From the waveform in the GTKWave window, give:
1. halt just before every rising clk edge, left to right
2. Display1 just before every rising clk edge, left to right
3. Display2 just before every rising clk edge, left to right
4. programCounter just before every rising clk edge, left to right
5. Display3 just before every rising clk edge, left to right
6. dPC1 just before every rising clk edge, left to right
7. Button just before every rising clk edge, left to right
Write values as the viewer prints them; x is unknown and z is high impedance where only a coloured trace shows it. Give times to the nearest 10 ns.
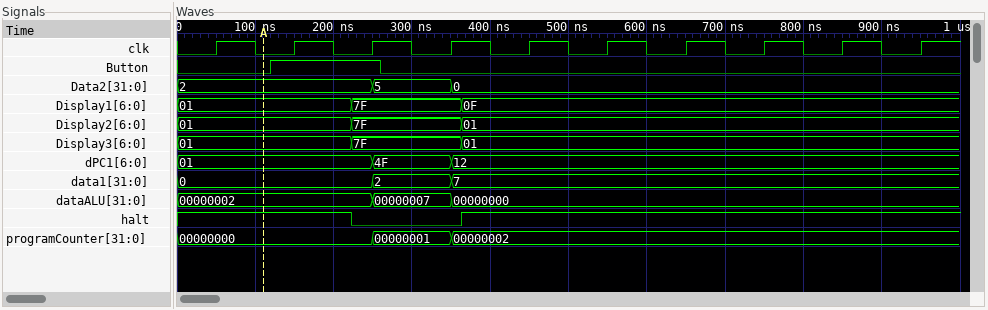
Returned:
1 1 0 0 1 1 1 1 1 1
01, 01, 7F, 7F, 0F, 0F, 0F, 0F, 0F, 0F
01, 01, 7F, 7F, 01, 01, 01, 01, 01, 01
00000000, 00000000, 00000000, 00000001, 00000002, 00000002, 00000002, 00000002, 00000002, 00000002
01, 01, 7F, 7F, 01, 01, 01, 01, 01, 01
01, 01, 01, 4F, 12, 12, 12, 12, 12, 12
0 1 1 0 0 0 0 0 0 0
